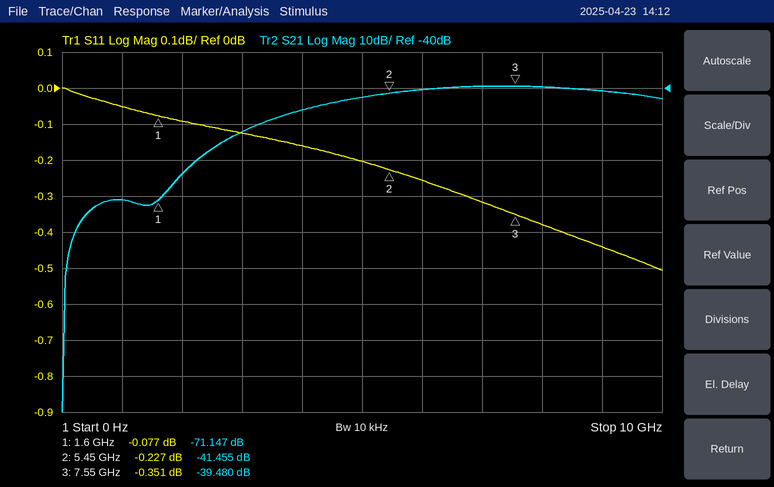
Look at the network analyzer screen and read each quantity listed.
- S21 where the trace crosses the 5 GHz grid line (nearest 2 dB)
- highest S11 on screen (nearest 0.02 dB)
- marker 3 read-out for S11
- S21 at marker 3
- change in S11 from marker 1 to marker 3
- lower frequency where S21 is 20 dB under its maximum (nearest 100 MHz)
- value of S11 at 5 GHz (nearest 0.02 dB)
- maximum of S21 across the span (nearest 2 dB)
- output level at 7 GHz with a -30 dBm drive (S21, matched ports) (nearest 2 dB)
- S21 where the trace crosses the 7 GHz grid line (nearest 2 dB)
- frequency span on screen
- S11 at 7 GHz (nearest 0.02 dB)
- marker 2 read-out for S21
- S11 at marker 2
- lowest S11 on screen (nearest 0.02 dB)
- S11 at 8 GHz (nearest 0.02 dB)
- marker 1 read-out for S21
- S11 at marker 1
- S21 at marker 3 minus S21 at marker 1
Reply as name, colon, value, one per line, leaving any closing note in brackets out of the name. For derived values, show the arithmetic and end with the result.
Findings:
S21 where the trace crosses the 5 GHz grid line: -42 dB
highest S11 on screen: 0.00 dB
marker 3 read-out for S11: -0.351 dB
S21 at marker 3: -39.480 dB
change in S11 from marker 1 to marker 3: -0.351 − (-0.077) = -0.274 dB
lower frequency where S21 is 20 dB under its maximum: 2.3 GHz
value of S11 at 5 GHz: -0.20 dB
maximum of S21 across the span: -40 dB
output level at 7 GHz with a -30 dBm drive (S21, matched ports): -30 dBm + (-40 dB) = -70 dBm
S21 where the trace crosses the 7 GHz grid line: -40 dB
frequency span on screen: 10 GHz
S11 at 7 GHz: -0.32 dB
marker 2 read-out for S21: -41.455 dB
S11 at marker 2: -0.227 dB
lowest S11 on screen: -0.50 dB
S11 at 8 GHz: -0.38 dB
marker 1 read-out for S21: -71.147 dB
S11 at marker 1: -0.077 dB
S21 at marker 3 minus S21 at marker 1: -39.48 − (-71.147) = 31.667 dB
